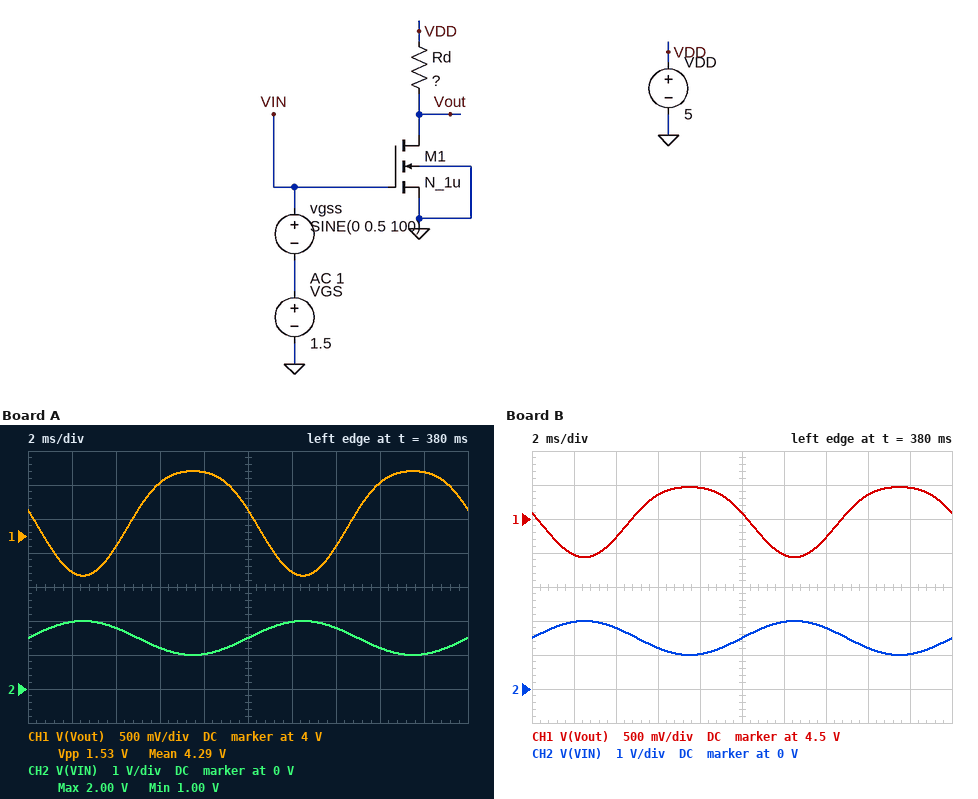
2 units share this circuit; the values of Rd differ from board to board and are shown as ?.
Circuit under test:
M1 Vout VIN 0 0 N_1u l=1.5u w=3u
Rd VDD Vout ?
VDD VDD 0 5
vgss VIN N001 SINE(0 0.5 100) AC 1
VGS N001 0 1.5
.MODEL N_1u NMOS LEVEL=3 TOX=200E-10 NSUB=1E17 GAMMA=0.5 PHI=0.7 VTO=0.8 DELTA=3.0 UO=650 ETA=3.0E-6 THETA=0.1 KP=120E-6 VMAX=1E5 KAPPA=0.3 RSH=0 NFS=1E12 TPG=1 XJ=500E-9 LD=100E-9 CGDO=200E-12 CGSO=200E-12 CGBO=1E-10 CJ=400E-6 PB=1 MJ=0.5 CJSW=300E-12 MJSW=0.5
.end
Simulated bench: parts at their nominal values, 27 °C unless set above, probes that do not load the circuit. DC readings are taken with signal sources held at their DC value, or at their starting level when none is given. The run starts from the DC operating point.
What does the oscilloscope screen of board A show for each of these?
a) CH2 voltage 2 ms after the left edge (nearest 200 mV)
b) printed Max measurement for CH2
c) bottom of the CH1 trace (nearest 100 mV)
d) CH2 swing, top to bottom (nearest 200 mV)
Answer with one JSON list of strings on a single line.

["2.0 V", "2.00 V", "3.4 V", "1.0 V"]
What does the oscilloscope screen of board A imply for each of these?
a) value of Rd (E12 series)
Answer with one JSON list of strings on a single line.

["15 kΩ"]
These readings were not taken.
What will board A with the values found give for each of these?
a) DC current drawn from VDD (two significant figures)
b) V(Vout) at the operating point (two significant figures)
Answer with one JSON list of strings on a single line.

["41 µA", "4.4 V"]
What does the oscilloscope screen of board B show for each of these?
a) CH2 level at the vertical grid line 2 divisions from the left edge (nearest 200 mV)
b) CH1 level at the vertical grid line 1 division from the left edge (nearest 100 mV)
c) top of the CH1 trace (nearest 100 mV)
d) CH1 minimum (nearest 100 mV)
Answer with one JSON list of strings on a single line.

["1.8 V", "4.0 V", "5.0 V", "3.9 V"]
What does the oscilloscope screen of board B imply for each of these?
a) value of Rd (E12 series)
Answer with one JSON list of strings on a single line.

["10 kΩ"]
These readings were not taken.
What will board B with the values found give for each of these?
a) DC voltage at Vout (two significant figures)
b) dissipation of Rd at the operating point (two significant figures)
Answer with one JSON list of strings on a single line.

["4.6 V", "17 µW"]
